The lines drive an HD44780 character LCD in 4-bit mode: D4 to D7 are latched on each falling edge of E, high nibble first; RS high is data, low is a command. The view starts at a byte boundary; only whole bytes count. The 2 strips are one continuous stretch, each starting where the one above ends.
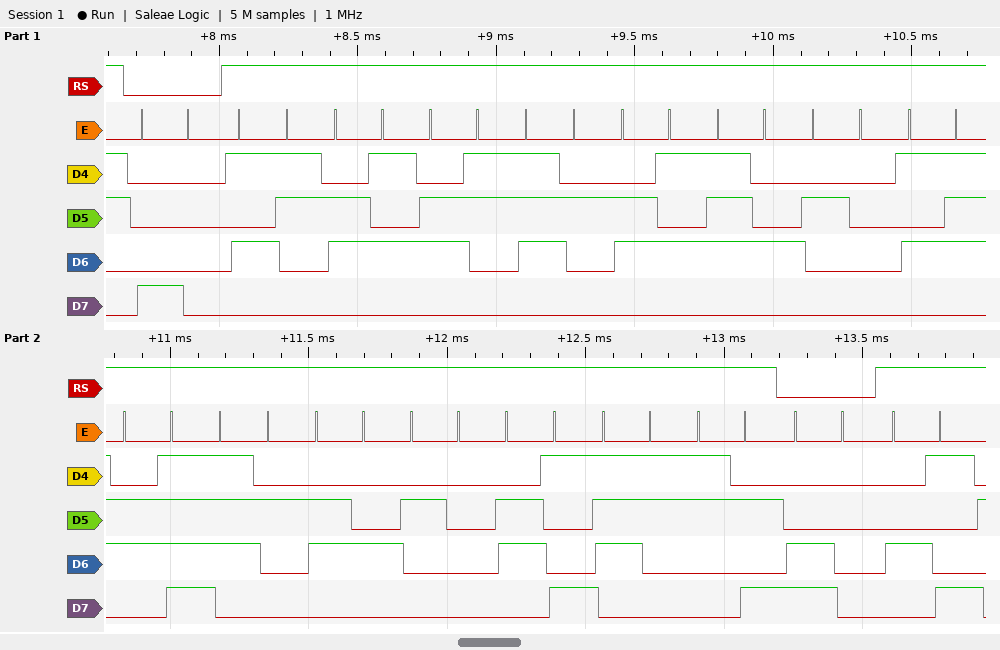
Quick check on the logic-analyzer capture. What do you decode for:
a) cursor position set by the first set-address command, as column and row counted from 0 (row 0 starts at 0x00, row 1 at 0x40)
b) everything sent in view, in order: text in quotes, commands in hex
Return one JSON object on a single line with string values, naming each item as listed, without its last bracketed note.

{"cursor position set by the first set-address command, as column and row counted from 0": "column 0, row 0", "everything sent in view, in order: text in quotes, commands in hex": "0x80 \"Secret Word is:\" 0xC0 \"I\""}
